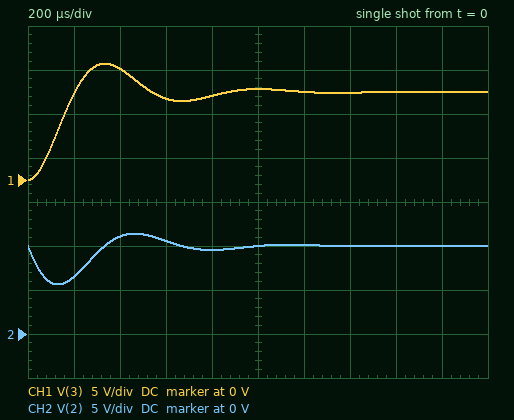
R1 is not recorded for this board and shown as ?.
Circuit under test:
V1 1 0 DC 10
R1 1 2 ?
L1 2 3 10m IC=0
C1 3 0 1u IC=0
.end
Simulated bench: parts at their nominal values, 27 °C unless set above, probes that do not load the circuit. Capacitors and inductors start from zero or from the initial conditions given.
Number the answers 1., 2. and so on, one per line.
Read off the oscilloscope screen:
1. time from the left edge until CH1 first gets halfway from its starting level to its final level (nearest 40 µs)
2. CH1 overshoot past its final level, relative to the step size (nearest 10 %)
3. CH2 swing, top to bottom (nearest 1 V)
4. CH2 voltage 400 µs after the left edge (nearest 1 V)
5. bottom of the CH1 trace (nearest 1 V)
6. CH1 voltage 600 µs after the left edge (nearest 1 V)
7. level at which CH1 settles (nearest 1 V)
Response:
1. 120 µs
2. 30 %
3. 6 V
4. 11 V
5. 0 V
6. 9 V
7. 10 V
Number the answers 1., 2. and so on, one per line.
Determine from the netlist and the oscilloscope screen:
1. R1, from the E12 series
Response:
1. 68 Ω
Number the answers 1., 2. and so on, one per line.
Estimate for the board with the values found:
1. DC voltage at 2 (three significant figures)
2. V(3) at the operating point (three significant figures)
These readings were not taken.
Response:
1. 10.0 V
2. 10.0 V
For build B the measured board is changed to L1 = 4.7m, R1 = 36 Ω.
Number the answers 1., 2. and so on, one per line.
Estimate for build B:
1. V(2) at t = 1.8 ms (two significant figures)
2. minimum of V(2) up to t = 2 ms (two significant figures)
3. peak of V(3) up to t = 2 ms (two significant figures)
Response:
1. 10 V
2. 6.3 V
3. 14 V
